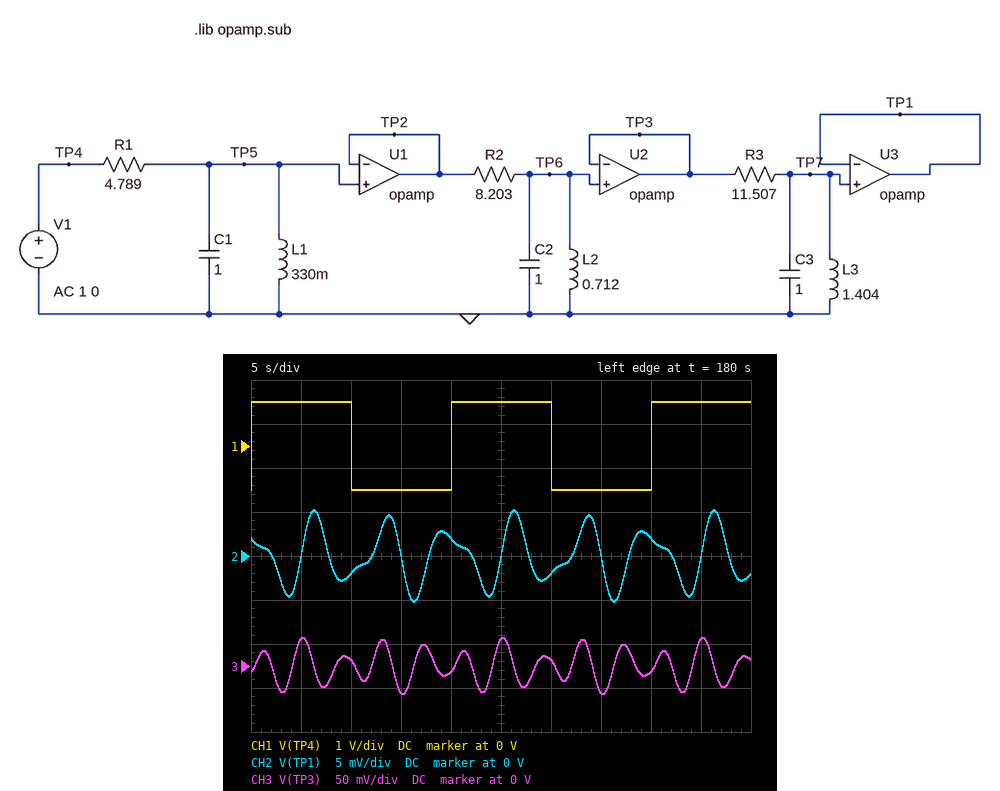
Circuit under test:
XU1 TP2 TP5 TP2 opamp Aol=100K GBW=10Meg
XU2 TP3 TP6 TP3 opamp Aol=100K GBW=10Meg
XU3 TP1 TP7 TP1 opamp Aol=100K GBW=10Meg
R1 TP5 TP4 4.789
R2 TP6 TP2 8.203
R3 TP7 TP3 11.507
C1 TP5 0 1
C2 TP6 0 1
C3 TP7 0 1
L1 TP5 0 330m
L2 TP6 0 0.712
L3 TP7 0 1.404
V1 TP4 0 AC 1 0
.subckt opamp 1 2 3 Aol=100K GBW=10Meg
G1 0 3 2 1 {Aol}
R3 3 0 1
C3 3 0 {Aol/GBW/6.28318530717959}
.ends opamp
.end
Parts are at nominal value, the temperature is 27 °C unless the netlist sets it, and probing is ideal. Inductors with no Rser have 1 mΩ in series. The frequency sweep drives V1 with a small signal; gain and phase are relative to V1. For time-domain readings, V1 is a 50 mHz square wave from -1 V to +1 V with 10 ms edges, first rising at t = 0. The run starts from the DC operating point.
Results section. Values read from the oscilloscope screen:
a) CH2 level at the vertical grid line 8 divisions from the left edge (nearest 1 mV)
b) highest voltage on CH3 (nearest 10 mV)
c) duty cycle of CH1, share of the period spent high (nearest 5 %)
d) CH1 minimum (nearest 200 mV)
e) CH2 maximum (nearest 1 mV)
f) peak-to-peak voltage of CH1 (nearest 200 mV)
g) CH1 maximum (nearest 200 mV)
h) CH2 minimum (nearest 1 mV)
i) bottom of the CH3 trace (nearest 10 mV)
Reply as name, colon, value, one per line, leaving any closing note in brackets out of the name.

CH2 level at the vertical grid line 8 divisions from the left edge: 2 mV
highest voltage on CH3: 30 mV
duty cycle of CH1, share of the period spent high: 50 %
CH1 minimum: -1.0 V
CH2 maximum: 5 mV
peak-to-peak voltage of CH1: 2.0 V
CH1 maximum: 1.0 V
CH2 minimum: -5 mV
bottom of the CH3 trace: -30 mV
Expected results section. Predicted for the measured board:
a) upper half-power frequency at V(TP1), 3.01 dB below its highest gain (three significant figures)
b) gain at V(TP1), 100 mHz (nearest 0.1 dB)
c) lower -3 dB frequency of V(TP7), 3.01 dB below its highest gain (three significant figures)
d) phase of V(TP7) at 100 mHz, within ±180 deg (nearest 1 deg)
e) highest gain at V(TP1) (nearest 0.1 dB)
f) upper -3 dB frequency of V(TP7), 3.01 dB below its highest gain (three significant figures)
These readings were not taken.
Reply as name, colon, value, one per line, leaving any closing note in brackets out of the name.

upper half-power frequency at V(TP1), 3.01 dB below its highest gain: 199 mHz
gain at V(TP1), 100 mHz: -63.9 dB
lower -3 dB frequency of V(TP7), 3.01 dB below its highest gain: 178 mHz
phase of V(TP7) at 100 mHz, within ±180 deg: -108 deg
highest gain at V(TP1): -33.2 dB
upper -3 dB frequency of V(TP7), 3.01 dB below its highest gain: 199 mHz
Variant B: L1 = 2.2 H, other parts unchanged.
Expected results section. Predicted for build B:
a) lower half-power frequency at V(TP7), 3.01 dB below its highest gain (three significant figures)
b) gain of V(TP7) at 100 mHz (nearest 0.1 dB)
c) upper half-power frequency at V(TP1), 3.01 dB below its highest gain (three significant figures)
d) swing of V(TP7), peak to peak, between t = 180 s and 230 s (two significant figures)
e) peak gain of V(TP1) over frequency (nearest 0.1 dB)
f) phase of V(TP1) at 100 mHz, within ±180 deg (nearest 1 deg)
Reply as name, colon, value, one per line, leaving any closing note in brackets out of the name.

lower half-power frequency at V(TP7), 3.01 dB below its highest gain: 127 mHz
gain of V(TP7) at 100 mHz: -38.7 dB
upper half-power frequency at V(TP1), 3.01 dB below its highest gain: 142 mHz
swing of V(TP7), peak to peak, between t = 180 s and 230 s: 33 mV
peak gain of V(TP1) over frequency: -21.7 dB
phase of V(TP1) at 100 mHz, within ±180 deg: -170 deg
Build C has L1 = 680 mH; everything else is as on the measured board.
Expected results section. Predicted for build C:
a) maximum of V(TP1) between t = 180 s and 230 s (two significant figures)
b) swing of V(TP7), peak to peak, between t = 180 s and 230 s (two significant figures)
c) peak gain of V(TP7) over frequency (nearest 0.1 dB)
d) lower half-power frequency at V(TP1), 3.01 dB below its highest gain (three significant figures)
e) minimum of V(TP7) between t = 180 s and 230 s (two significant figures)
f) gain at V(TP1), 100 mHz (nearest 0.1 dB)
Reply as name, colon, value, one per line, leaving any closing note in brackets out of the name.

maximum of V(TP1) between t = 180 s and 230 s: 13 mV
swing of V(TP7), peak to peak, between t = 180 s and 230 s: 27 mV
peak gain of V(TP7) over frequency: -17.1 dB
lower half-power frequency at V(TP1), 3.01 dB below its highest gain: 180 mHz
minimum of V(TP7) between t = 180 s and 230 s: -13 mV
gain at V(TP1), 100 mHz: -56.2 dB
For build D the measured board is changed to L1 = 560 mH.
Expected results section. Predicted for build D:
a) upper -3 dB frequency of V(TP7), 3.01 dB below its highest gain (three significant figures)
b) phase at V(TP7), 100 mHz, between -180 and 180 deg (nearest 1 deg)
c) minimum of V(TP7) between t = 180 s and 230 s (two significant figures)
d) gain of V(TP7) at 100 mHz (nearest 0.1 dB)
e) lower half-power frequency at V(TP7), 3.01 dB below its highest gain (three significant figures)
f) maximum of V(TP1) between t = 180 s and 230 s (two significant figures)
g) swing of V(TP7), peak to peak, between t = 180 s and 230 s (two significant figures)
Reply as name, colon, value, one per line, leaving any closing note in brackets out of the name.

upper -3 dB frequency of V(TP7), 3.01 dB below its highest gain: 204 mHz
phase at V(TP7), 100 mHz, between -180 and 180 deg: -110 deg
minimum of V(TP7) between t = 180 s and 230 s: -9.6 mV
gain of V(TP7) at 100 mHz: -58.4 dB
lower half-power frequency at V(TP7), 3.01 dB below its highest gain: 181 mHz
maximum of V(TP1) between t = 180 s and 230 s: 9.6 mV
swing of V(TP7), peak to peak, between t = 180 s and 230 s: 19 mV
